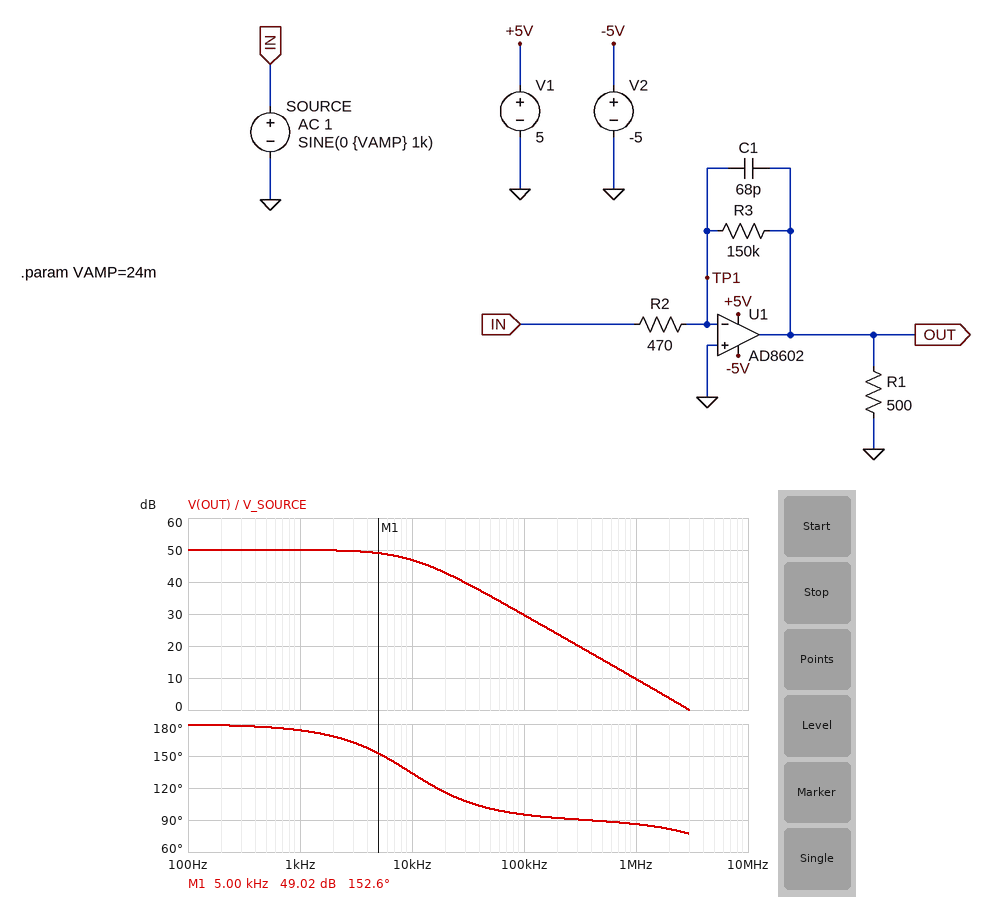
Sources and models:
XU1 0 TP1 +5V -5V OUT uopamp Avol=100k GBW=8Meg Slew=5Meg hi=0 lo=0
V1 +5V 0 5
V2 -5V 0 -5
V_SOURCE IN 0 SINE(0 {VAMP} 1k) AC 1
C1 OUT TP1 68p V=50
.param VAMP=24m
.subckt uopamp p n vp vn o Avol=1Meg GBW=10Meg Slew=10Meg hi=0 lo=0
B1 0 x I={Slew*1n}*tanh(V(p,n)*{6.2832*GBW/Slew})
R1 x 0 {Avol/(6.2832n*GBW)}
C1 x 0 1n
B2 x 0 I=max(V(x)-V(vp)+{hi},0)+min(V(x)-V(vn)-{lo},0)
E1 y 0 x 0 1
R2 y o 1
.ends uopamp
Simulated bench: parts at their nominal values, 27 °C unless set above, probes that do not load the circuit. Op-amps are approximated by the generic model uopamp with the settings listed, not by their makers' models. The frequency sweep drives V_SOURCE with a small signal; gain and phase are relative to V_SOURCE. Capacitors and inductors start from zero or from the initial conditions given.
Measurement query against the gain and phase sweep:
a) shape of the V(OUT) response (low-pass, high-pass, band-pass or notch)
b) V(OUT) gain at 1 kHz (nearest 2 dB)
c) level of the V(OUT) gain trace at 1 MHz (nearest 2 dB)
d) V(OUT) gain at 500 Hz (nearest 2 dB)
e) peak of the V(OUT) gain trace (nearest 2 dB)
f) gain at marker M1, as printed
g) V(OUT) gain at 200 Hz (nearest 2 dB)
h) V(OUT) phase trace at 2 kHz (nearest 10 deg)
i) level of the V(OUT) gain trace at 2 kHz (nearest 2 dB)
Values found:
low-pass
50 dB
10 dB
50 dB
50 dB
49.02 dB
50 dB
170 deg
50 dB
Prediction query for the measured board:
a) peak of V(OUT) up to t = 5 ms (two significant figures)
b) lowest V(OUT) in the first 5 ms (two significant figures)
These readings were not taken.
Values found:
5.0 V
-5.0 V
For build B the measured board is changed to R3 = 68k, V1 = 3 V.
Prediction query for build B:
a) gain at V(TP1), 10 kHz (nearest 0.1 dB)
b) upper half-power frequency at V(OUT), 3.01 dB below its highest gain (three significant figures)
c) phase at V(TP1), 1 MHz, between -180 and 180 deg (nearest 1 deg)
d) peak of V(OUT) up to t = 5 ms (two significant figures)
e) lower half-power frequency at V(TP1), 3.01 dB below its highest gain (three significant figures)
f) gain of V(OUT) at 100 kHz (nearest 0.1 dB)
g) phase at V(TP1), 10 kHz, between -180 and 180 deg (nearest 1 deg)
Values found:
-15.7 dB
21.2 kHz
-3 deg
3.0 V
21.1 kHz
29.5 dB
64 deg
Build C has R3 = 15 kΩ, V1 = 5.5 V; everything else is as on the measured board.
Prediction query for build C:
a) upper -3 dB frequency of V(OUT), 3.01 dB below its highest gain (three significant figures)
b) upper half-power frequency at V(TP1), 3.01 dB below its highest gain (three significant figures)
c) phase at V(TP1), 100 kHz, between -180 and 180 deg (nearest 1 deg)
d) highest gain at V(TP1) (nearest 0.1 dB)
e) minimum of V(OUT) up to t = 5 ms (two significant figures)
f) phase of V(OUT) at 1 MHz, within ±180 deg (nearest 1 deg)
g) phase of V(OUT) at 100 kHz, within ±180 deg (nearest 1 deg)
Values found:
95.7 kHz
13.2 MHz
43 deg
-8.4 dB
-770 mV
91 deg
133 deg
